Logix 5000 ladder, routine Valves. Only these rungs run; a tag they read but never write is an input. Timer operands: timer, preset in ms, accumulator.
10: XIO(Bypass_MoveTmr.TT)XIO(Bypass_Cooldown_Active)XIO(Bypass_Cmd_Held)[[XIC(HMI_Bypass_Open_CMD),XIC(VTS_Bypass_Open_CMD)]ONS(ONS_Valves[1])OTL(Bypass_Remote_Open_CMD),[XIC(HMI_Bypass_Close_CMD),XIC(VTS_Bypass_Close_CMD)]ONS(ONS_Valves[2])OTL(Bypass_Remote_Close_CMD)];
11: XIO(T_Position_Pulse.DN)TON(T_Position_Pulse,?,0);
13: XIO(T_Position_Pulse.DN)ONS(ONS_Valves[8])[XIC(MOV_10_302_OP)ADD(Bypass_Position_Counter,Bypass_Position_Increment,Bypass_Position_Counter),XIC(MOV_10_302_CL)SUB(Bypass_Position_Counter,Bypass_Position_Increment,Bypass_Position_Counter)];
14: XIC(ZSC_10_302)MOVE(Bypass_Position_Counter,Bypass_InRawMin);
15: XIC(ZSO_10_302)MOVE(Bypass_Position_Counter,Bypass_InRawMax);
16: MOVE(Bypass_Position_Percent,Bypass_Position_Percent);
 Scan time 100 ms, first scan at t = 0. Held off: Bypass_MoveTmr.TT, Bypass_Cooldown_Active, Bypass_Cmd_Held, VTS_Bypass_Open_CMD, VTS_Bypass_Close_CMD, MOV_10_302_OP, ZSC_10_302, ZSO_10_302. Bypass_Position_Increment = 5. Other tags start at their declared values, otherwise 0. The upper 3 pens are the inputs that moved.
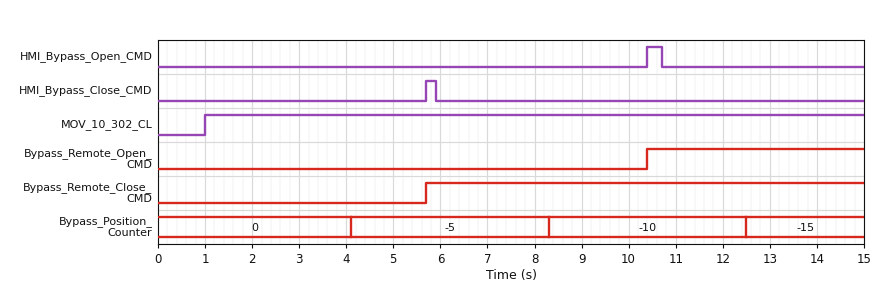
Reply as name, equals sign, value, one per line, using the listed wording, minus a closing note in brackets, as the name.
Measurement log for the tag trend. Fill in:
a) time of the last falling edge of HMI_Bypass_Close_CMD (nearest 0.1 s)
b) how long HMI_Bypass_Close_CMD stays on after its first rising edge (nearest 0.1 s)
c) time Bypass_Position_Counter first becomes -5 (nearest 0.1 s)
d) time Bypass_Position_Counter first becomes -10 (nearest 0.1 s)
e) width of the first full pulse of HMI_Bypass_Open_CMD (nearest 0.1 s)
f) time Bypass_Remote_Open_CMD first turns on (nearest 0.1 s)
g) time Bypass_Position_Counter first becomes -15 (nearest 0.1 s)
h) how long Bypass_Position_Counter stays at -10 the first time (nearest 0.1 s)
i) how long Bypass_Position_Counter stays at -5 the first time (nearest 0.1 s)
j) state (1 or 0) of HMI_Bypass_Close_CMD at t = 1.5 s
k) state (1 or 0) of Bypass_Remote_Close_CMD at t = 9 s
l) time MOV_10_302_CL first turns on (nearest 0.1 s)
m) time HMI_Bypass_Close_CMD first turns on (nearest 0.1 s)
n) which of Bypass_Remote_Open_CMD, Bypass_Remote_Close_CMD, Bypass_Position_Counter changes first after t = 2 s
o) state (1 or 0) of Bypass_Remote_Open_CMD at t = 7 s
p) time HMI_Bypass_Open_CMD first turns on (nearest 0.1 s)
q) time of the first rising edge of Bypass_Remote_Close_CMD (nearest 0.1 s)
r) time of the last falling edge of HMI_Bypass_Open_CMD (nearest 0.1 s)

time of the last falling edge of HMI_Bypass_Close_CMD = 5.9 s
how long HMI_Bypass_Close_CMD stays on after its first rising edge = 0.2 s
time Bypass_Position_Counter first becomes -5 = 4.1 s
time Bypass_Position_Counter first becomes -10 = 8.3 s
width of the first full pulse of HMI_Bypass_Open_CMD = 0.3 s
time Bypass_Remote_Open_CMD first turns on = 10.4 s
time Bypass_Position_Counter first becomes -15 = 12.5 s
how long Bypass_Position_Counter stays at -10 the first time = 4.2 s
how long Bypass_Position_Counter stays at -5 the first time = 4.2 s
state (1 or 0) of HMI_Bypass_Close_CMD at t = 1.5 s = 0
state (1 or 0) of Bypass_Remote_Close_CMD at t = 9 s = 1
time MOV_10_302_CL first turns on = 1.0 s
time HMI_Bypass_Close_CMD first turns on = 5.7 s
which of Bypass_Remote_Open_CMD, Bypass_Remote_Close_CMD, Bypass_Position_Counter changes first after t = 2 s = Bypass_Position_Counter
state (1 or 0) of Bypass_Remote_Open_CMD at t = 7 s = 0
time HMI_Bypass_Open_CMD first turns on = 10.4 s
time of the first rising edge of Bypass_Remote_Close_CMD = 5.7 s
time of the last falling edge of HMI_Bypass_Open_CMD = 10.7 s
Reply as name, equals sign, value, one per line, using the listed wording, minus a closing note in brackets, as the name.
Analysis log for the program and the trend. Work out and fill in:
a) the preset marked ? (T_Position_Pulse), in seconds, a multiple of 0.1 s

the preset marked ? (T_Position_Pulse), in seconds, a multiple of 0.1 s = 4.0 s
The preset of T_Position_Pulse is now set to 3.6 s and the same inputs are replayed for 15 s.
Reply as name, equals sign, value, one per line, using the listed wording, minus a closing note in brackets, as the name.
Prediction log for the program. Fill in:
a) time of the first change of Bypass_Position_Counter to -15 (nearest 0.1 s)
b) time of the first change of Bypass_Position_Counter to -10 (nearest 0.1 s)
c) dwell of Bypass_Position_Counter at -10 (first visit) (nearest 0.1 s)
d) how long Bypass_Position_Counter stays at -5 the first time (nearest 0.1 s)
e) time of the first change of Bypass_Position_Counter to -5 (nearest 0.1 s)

time of the first change of Bypass_Position_Counter to -15 = 11.3 s
time of the first change of Bypass_Position_Counter to -10 = 7.5 s
dwell of Bypass_Position_Counter at -10 (first visit) = 3.8 s
how long Bypass_Position_Counter stays at -5 the first time = 3.8 s
time of the first change of Bypass_Position_Counter to -5 = 3.7 s
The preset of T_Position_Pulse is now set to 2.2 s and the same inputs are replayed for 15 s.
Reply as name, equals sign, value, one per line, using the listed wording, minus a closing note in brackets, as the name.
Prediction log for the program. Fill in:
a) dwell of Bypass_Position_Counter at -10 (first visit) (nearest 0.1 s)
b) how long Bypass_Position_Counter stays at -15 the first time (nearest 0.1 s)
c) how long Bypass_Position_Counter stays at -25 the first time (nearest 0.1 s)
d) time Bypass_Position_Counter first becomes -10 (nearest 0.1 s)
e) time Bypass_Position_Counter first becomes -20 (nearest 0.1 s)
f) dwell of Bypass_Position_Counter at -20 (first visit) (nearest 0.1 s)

dwell of Bypass_Position_Counter at -10 (first visit) = 2.4 s
how long Bypass_Position_Counter stays at -15 the first time = 2.4 s
how long Bypass_Position_Counter stays at -25 the first time = 2.4 s
time Bypass_Position_Counter first becomes -10 = 4.7 s
time Bypass_Position_Counter first becomes -20 = 9.5 s
dwell of Bypass_Position_Counter at -20 (first visit) = 2.4 s
